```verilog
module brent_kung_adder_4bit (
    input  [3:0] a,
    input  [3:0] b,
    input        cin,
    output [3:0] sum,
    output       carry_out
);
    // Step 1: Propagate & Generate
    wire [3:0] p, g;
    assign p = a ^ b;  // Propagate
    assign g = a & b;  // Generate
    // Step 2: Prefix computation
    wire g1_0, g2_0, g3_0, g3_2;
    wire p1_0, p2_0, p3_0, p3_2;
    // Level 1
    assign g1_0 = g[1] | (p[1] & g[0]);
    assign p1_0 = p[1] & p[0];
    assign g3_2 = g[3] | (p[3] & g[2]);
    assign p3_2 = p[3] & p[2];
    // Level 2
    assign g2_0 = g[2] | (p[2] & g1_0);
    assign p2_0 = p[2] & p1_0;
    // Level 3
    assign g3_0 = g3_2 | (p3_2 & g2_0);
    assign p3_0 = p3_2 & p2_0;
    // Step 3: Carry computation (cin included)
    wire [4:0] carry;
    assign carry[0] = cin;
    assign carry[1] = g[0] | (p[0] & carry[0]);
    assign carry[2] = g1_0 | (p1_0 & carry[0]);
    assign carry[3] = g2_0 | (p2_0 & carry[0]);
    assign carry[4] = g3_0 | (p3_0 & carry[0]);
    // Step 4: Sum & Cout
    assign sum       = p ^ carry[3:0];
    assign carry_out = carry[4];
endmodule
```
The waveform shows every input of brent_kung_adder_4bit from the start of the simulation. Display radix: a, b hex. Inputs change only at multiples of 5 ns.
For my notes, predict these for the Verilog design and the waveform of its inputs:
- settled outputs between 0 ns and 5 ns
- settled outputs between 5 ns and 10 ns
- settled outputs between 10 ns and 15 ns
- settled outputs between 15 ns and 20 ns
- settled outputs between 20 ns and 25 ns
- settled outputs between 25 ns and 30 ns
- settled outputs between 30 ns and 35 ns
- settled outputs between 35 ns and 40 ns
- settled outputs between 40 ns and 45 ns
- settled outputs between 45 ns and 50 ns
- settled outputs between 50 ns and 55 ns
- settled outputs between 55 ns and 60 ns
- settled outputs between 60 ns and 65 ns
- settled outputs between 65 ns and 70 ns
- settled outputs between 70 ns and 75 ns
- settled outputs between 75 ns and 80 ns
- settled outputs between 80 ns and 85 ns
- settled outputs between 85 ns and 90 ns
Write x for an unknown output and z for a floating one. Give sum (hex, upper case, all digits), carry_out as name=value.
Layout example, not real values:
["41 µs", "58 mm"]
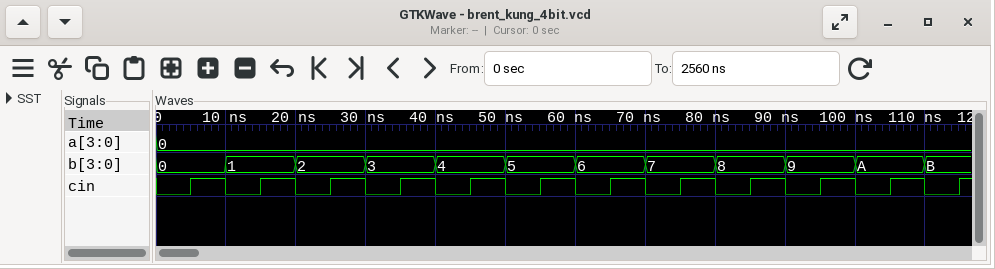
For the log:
["sum=0, carry_out=0", "sum=1, carry_out=0", "sum=1, carry_out=0", "sum=2, carry_out=0", "sum=2, carry_out=0", "sum=3, carry_out=0", "sum=3, carry_out=0", "sum=4, carry_out=0", "sum=4, carry_out=0", "sum=5, carry_out=0", "sum=5, carry_out=0", "sum=6, carry_out=0", "sum=6, carry_out=0", "sum=7, carry_out=0", "sum=7, carry_out=0", "sum=8, carry_out=0", "sum=8, carry_out=0", "sum=9, carry_out=0"]
